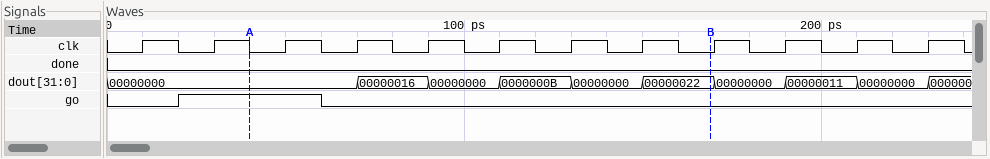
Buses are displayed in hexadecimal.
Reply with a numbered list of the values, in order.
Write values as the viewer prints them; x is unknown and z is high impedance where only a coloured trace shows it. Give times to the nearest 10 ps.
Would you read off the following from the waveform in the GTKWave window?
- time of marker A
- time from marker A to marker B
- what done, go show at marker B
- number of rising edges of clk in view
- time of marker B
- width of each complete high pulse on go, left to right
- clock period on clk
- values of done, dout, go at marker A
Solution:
1. 40 ps
2. 130 ps
3. done=0, go=0
4. 12
5. 170 ps
6. 40 ps
7. 20 ps
8. done=0, dout=00000000, go=1
